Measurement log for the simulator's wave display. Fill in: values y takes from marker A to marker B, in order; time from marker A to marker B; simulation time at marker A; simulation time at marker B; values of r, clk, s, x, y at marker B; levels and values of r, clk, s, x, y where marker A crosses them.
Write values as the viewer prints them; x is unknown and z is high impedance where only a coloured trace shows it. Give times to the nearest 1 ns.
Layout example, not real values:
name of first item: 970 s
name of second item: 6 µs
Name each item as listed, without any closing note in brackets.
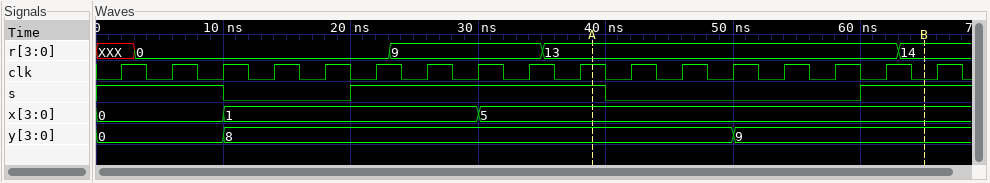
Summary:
values y takes from marker A to marker B, in order: 8, 9
time from marker A to marker B: 26 ns
simulation time at marker A: 39 ns
simulation time at marker B: 65 ns
values of r, clk, s, x, y at marker B: r=14, clk=0, s=1, x=5, y=9
levels and values of r, clk, s, x, y where marker A crosses them: r=13, clk=1, s=1, x=5, y=8
